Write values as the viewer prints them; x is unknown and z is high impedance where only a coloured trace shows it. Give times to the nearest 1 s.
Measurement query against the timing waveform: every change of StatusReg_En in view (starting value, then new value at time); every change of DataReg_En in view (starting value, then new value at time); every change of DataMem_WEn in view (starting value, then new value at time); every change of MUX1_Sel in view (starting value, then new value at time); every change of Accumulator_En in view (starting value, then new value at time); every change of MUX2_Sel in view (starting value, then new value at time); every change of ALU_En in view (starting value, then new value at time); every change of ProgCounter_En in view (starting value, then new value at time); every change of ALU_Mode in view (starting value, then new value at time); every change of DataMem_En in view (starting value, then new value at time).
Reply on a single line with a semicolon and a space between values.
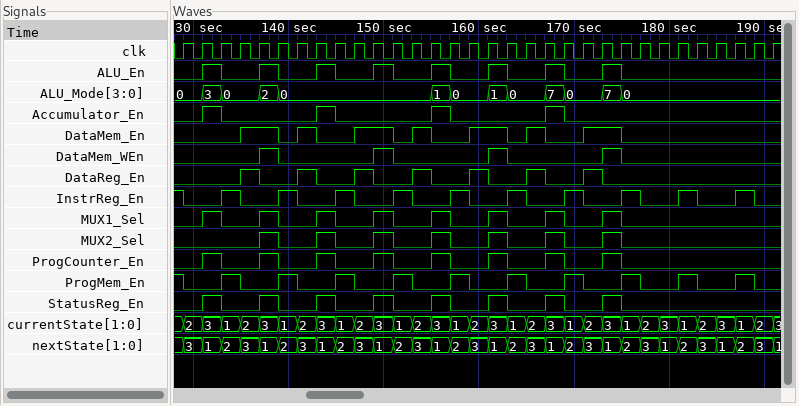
0, 1 at 131 s, 0 at 133 s, 1 at 137 s, 0 at 139 s, 1 at 143 s, 0 at 145 s, 1 at 149 s, 0 at 151 s, 1 at 155 s, 0 at 157 s, 1 at 161 s, 0 at 163 s, 1 at 167 s, 0 at 169 s, 1 at 173 s, 0 at 175 s; 0, 1 at 135 s, 0 at 137 s, 1 at 141 s, 0 at 143 s, 1 at 147 s, 0 at 149 s, 1 at 153 s, 0 at 155 s, 1 at 159 s, 0 at 161 s, 1 at 165 s, 0 at 167 s, 1 at 171 s, 0 at 173 s; 0, 1 at 137 s, 0 at 139 s, 1 at 149 s, 0 at 151 s, 1 at 161 s, 0 at 163 s, 1 at 173 s, 0 at 175 s; 0, 1 at 131 s, 0 at 133 s, 1 at 137 s, 0 at 139 s, 1 at 143 s, 0 at 145 s, 1 at 149 s, 0 at 151 s, 1 at 155 s, 0 at 157 s, 1 at 161 s, 0 at 163 s, 1 at 167 s, 0 at 169 s, 1 at 173 s, 0 at 175 s; 0, 1 at 131 s, 0 at 133 s, 1 at 143 s, 0 at 145 s, 1 at 155 s, 0 at 157 s, 1 at 167 s, 0 at 169 s; 0, 1 at 137 s, 0 at 139 s, 1 at 143 s, 0 at 145 s, 1 at 149 s, 0 at 151 s, 1 at 155 s, 0 at 157 s, 1 at 161 s, 0 at 163 s, 1 at 167 s, 0 at 169 s, 1 at 173 s, 0 at 175 s; 0, 1 at 131 s, 0 at 133 s, 1 at 137 s, 0 at 139 s, 1 at 143 s, 0 at 145 s, 1 at 149 s, 0 at 151 s, 1 at 155 s, 0 at 157 s, 1 at 161 s, 0 at 163 s, 1 at 167 s, 0 at 169 s, 1 at 173 s, 0 at 175 s; 0, 1 at 131 s, 0 at 133 s, 1 at 137 s, 0 at 139 s, 1 at 143 s, 0 at 145 s, 1 at 149 s, 0 at 151 s, 1 at 155 s, 0 at 157 s, 1 at 161 s, 0 at 163 s, 1 at 167 s, 0 at 169 s, 1 at 173 s, 0 at 175 s; 0, 3 at 131 s, 0 at 133 s, 2 at 137 s, 0 at 139 s, 1 at 155 s, 0 at 157 s, 1 at 161 s, 0 at 163 s, 7 at 167 s, 0 at 169 s, 7 at 173 s, 0 at 175 s; 0, 1 at 135 s, 0 at 139 s, 1 at 141 s, 0 at 143 s, 1 at 147 s, 0 at 151 s, 1 at 153 s, 0 at 155 s, 1 at 159 s, 0 at 163 s, 1 at 165 s, 0 at 167 s, 1 at 171 s, 0 at 175 s
